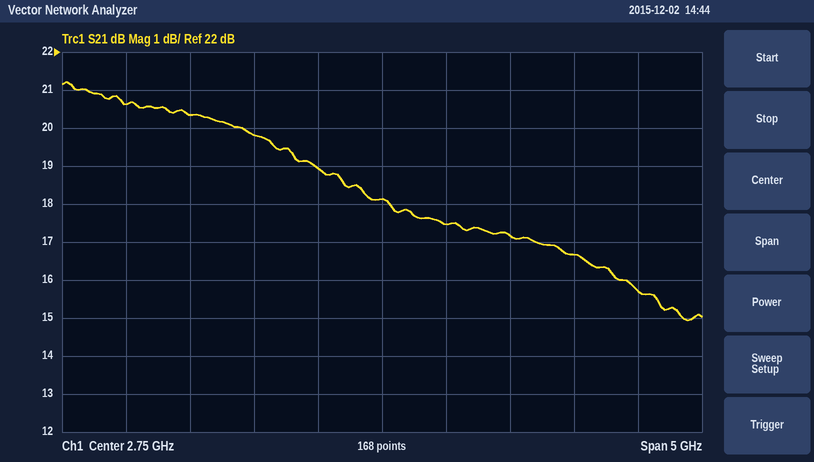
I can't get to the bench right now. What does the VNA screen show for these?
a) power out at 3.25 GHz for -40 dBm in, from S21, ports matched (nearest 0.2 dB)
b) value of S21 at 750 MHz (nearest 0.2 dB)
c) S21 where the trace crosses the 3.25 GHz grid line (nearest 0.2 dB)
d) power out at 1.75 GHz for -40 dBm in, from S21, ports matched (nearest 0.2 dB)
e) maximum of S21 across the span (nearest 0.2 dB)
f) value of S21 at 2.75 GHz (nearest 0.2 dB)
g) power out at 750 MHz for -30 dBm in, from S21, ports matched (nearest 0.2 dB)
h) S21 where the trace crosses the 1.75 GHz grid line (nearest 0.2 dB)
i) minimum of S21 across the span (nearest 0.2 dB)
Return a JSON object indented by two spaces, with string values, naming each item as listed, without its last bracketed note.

{
  "power out at 3.25 GHz for -40 dBm in, from S21, ports matched": "-22.6 dBm",
  "value of S21 at 750 MHz": "20.6 dB",
  "S21 where the trace crosses the 3.25 GHz grid line": "17.4 dB",
  "power out at 1.75 GHz for -40 dBm in, from S21, ports matched": "-20.2 dBm",
  "maximum of S21 across the span": "21.2 dB",
  "value of S21 at 2.75 GHz": "18.2 dB",
  "power out at 750 MHz for -30 dBm in, from S21, ports matched": "-9.4 dBm",
  "S21 where the trace crosses the 1.75 GHz grid line": "19.8 dB",
  "minimum of S21 across the span": "15.0 dB"
}
